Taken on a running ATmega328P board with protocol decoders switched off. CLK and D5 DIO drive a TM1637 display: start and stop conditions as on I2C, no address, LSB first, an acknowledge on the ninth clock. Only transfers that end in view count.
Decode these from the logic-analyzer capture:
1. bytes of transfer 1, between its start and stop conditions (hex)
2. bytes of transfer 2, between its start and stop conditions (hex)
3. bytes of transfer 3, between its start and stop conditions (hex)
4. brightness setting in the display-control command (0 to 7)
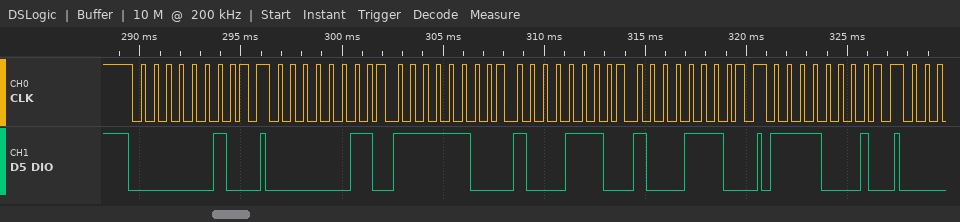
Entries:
40
C0 3F 71 71
8F
7
